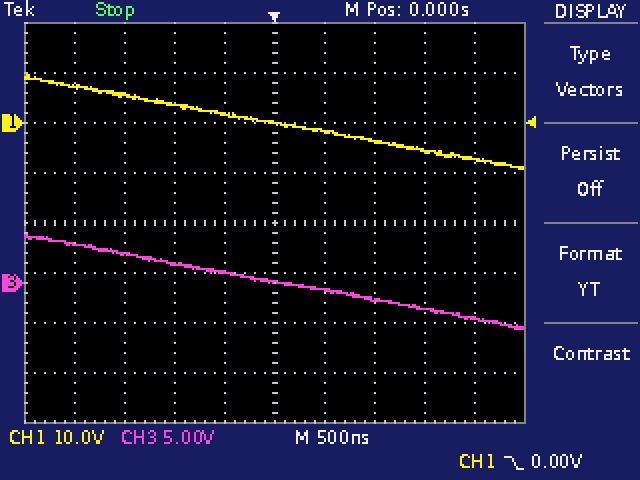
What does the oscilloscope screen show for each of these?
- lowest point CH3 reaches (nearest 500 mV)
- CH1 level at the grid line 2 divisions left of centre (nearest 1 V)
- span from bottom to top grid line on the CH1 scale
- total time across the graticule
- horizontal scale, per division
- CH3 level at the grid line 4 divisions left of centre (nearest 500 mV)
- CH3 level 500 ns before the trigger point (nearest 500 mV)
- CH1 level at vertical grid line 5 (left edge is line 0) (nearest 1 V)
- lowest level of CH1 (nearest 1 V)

-4.5 V
4 V
80 V
5 µs
500 ns
4.0 V
1.0 V
0 V
-9 V
